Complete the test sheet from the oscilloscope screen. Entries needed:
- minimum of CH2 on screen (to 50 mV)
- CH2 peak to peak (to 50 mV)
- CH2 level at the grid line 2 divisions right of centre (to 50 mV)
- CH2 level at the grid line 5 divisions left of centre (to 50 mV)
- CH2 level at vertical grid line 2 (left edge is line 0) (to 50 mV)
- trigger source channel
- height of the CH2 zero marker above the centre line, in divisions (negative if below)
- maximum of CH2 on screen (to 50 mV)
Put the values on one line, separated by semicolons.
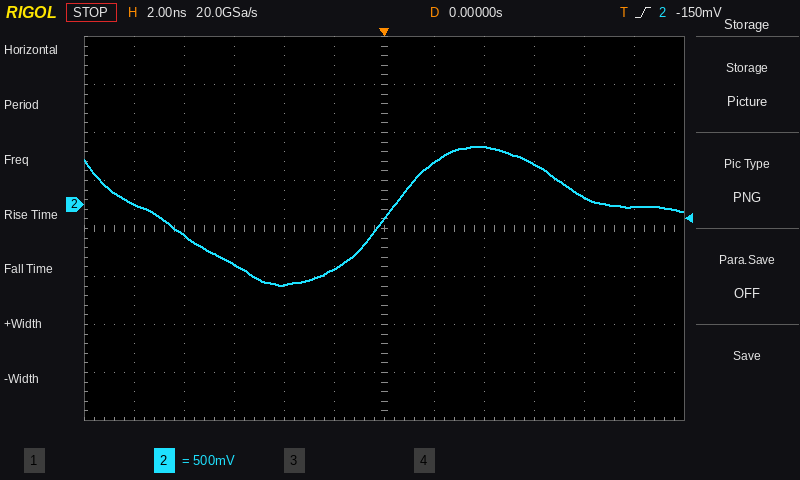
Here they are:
-850 mV; 1.45 V; 600 mV; 0 mV; -300 mV; CH2; +0.5 div; 600 mV
